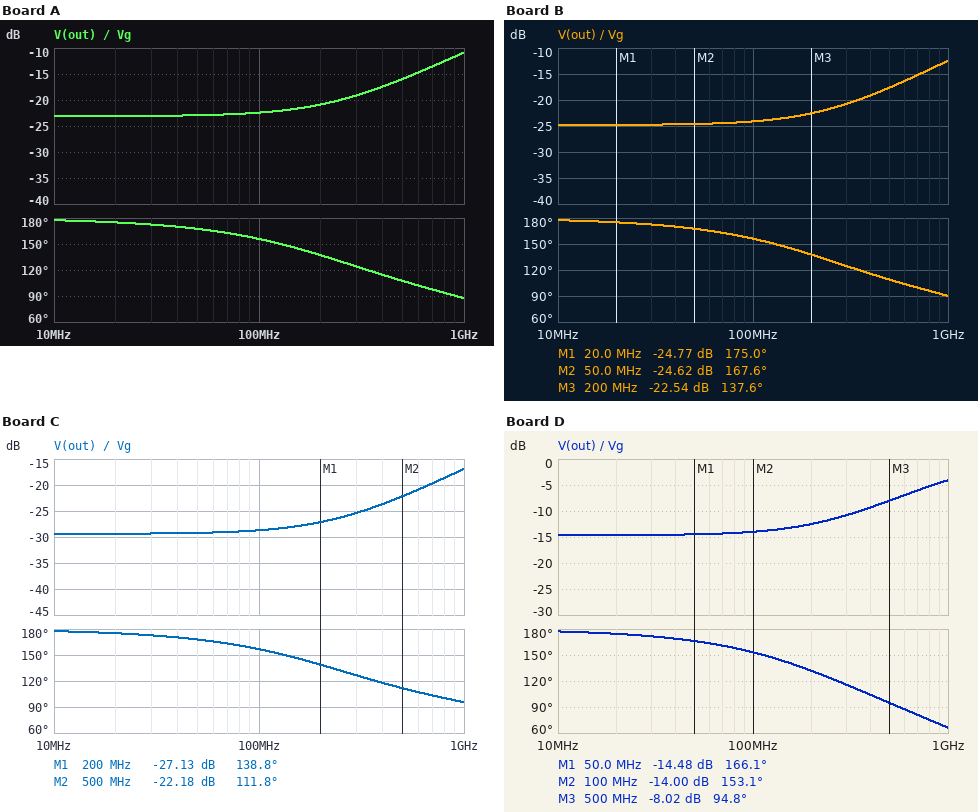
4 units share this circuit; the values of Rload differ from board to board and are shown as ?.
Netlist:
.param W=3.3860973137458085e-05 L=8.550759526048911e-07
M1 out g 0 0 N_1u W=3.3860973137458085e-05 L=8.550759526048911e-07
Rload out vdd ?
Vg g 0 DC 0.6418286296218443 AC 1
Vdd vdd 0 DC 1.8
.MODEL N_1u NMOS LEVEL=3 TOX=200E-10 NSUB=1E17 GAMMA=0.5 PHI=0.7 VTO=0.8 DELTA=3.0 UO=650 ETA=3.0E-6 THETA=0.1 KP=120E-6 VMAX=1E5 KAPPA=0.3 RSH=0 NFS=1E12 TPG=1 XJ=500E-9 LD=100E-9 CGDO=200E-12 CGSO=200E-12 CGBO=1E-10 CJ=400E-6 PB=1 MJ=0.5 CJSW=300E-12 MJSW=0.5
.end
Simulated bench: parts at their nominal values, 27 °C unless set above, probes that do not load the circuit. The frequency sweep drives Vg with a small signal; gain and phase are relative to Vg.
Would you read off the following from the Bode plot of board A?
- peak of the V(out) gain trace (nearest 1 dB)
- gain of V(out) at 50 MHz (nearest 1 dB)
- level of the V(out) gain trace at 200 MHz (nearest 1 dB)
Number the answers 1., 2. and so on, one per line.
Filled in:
1. -11 dB
2. -23 dB
3. -21 dB
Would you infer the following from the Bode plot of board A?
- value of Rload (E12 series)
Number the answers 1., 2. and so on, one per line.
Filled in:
1. 6.8 kΩ
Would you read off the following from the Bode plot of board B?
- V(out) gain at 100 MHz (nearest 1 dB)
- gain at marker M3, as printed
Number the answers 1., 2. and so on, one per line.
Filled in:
1. -24 dB
2. -22.54 dB
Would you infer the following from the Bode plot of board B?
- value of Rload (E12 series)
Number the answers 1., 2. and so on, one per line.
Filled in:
1. 5.6 kΩ
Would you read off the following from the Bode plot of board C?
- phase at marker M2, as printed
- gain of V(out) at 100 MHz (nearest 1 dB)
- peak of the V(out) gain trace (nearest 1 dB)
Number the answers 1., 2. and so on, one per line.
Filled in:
1. 111.8 deg
2. -29 dB
3. -17 dB
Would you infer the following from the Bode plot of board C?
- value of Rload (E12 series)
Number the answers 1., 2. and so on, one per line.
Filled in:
1. 3.3 kΩ
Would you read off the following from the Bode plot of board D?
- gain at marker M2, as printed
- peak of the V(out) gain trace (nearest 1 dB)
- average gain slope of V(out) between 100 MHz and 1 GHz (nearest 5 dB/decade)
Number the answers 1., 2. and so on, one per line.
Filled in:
1. -14.00 dB
2. -4 dB
3. 10 dB/decade
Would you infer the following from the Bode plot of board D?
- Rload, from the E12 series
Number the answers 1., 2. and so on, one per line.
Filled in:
1. 18 kΩ
